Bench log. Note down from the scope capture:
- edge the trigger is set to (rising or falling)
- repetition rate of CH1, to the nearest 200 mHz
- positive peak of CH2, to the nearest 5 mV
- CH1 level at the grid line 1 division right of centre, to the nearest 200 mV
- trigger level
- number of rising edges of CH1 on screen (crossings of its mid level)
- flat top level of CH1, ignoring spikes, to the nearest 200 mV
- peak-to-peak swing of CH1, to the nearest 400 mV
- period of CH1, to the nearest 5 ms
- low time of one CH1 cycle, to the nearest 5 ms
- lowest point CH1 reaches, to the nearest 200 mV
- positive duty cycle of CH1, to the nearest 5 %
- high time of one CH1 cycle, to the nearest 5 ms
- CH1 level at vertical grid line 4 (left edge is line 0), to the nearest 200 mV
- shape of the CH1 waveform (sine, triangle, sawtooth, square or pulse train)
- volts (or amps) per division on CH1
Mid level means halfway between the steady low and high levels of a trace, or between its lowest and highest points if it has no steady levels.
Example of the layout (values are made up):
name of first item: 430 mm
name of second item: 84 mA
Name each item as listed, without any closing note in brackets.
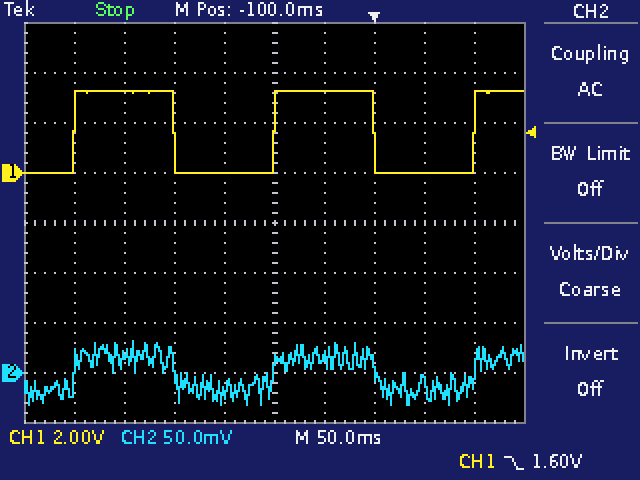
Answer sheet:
edge the trigger is set to: falling
repetition rate of CH1, to the nearest 200 mHz: 5.0 Hz
positive peak of CH2, to the nearest 5 mV: 30 mV
CH1 level at the grid line 1 division right of centre, to the nearest 200 mV: 3.2 V
trigger level: 1.60 V
number of rising edges of CH1 on screen: 3
flat top level of CH1, ignoring spikes, to the nearest 200 mV: 3.2 V
peak-to-peak swing of CH1, to the nearest 400 mV: 3.2 V
period of CH1, to the nearest 5 ms: 200 ms
low time of one CH1 cycle, to the nearest 5 ms: 100 ms
lowest point CH1 reaches, to the nearest 200 mV: 0.0 V
positive duty cycle of CH1, to the nearest 5 %: 50 %
high time of one CH1 cycle, to the nearest 5 ms: 100 ms
CH1 level at vertical grid line 4 (left edge is line 0), to the nearest 200 mV: 0.0 V
shape of the CH1 waveform: square
volts (or amps) per division on CH1: 2 V
